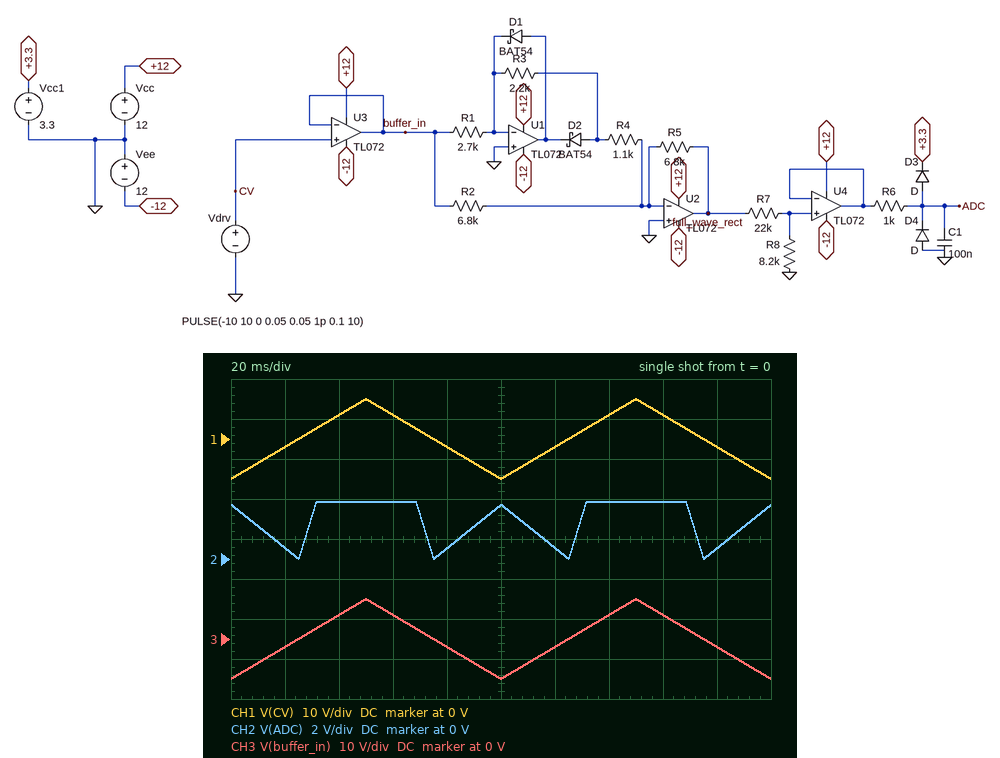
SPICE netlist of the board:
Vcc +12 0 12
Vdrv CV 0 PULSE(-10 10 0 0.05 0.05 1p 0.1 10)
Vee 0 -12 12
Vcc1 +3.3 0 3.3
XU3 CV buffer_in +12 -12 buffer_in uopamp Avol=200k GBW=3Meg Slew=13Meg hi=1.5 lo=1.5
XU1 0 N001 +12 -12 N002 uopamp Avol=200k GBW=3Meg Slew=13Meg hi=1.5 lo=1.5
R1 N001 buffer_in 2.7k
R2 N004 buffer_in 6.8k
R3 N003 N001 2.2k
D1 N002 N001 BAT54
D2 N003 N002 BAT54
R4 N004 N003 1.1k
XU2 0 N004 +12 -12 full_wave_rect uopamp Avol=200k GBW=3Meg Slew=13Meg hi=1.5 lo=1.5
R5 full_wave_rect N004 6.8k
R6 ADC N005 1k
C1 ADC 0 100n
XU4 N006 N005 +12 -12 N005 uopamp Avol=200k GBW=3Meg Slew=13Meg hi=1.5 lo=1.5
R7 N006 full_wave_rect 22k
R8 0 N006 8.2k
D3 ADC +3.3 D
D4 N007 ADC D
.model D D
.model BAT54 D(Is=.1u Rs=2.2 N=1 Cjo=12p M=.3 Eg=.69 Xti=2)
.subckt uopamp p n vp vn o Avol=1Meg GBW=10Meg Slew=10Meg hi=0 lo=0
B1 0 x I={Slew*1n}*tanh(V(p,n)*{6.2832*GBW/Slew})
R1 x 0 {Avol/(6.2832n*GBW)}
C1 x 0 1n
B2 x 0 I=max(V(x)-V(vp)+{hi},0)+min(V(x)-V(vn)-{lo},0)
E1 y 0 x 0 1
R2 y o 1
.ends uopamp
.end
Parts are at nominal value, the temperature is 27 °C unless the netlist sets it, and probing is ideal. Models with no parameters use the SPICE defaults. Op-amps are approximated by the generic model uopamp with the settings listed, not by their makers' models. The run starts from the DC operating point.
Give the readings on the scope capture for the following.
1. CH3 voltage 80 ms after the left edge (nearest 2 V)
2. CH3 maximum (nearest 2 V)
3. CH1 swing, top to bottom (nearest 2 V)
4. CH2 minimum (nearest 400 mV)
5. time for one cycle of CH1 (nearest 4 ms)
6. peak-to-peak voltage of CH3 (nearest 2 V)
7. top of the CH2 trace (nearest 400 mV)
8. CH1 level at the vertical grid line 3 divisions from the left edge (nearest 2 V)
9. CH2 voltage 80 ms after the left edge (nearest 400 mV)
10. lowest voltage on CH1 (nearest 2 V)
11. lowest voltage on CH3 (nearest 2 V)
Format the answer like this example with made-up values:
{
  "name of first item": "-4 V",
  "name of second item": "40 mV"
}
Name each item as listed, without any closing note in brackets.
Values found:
{
  "CH3 voltage 80 ms after the left edge": "-2 V",
  "CH3 maximum": "10 V",
  "CH1 swing, top to bottom": "20 V",
  "CH2 minimum": "0 V",
  "time for one cycle of CH1": "100 ms",
  "peak-to-peak voltage of CH3": "20 V",
  "top of the CH2 trace": "2.8 V",
  "CH1 level at the vertical grid line 3 divisions from the left edge": "6 V",
  "CH2 voltage 80 ms after the left edge": "400 mV",
  "lowest voltage on CH1": "-10 V",
  "lowest voltage on CH3": "-10 V"
}
